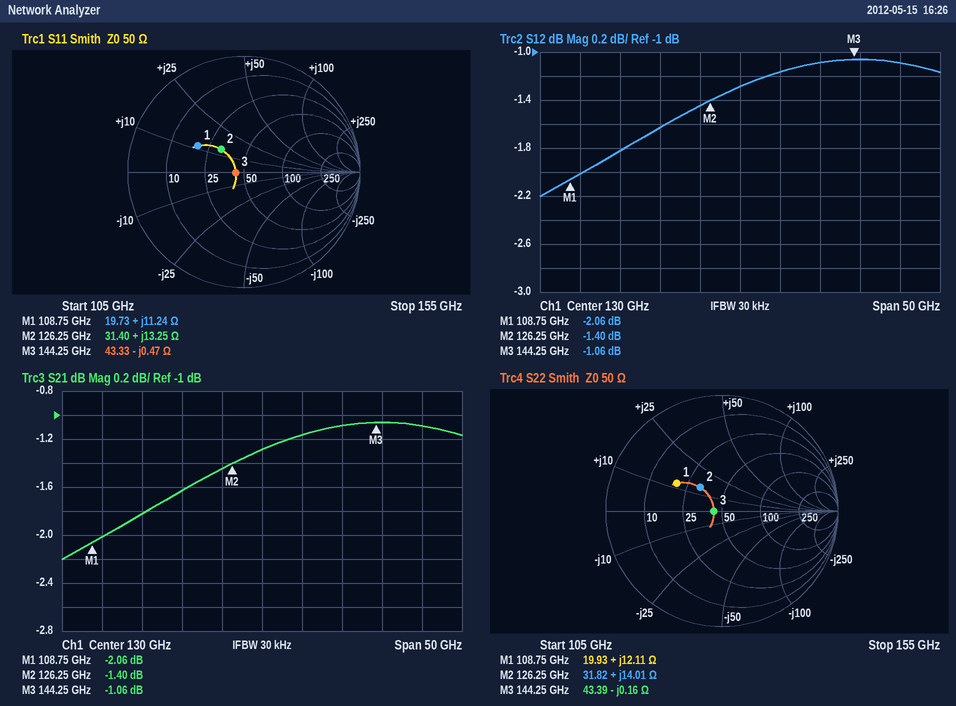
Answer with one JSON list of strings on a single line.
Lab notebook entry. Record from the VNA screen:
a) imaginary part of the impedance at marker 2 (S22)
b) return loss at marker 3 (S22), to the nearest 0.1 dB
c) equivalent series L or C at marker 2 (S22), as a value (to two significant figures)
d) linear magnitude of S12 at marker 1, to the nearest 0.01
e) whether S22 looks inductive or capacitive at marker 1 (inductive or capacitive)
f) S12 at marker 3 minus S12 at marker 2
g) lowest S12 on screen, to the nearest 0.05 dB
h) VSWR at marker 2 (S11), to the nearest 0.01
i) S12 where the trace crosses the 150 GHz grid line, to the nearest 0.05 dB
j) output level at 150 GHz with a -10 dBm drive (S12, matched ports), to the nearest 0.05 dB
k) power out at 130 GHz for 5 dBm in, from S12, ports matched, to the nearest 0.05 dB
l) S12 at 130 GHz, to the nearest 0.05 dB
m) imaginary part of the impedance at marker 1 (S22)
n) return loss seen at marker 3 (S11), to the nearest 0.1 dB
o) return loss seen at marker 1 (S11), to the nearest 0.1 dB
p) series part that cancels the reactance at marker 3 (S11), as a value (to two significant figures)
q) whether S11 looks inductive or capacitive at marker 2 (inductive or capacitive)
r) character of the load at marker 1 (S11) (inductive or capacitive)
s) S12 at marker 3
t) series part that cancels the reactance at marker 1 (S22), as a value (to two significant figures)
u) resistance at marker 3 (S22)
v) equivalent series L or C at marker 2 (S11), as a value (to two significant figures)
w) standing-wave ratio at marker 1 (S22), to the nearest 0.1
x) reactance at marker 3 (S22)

["+14.01 Ω", "23.0 dB", "18 pH", "0.79", "inductive", "0.34 dB", "-2.20 dB", "1.77", "-1.10 dB", "-11.10 dBm", "3.70 dBm", "-1.30 dB", "+12.11 Ω", "22.9 dB", "6.8 dB", "520 fH", "inductive", "inductive", "-1.06 dB", "120 fF", "43.39 Ω", "17 pH", "2.7", "-0.16 Ω"]
